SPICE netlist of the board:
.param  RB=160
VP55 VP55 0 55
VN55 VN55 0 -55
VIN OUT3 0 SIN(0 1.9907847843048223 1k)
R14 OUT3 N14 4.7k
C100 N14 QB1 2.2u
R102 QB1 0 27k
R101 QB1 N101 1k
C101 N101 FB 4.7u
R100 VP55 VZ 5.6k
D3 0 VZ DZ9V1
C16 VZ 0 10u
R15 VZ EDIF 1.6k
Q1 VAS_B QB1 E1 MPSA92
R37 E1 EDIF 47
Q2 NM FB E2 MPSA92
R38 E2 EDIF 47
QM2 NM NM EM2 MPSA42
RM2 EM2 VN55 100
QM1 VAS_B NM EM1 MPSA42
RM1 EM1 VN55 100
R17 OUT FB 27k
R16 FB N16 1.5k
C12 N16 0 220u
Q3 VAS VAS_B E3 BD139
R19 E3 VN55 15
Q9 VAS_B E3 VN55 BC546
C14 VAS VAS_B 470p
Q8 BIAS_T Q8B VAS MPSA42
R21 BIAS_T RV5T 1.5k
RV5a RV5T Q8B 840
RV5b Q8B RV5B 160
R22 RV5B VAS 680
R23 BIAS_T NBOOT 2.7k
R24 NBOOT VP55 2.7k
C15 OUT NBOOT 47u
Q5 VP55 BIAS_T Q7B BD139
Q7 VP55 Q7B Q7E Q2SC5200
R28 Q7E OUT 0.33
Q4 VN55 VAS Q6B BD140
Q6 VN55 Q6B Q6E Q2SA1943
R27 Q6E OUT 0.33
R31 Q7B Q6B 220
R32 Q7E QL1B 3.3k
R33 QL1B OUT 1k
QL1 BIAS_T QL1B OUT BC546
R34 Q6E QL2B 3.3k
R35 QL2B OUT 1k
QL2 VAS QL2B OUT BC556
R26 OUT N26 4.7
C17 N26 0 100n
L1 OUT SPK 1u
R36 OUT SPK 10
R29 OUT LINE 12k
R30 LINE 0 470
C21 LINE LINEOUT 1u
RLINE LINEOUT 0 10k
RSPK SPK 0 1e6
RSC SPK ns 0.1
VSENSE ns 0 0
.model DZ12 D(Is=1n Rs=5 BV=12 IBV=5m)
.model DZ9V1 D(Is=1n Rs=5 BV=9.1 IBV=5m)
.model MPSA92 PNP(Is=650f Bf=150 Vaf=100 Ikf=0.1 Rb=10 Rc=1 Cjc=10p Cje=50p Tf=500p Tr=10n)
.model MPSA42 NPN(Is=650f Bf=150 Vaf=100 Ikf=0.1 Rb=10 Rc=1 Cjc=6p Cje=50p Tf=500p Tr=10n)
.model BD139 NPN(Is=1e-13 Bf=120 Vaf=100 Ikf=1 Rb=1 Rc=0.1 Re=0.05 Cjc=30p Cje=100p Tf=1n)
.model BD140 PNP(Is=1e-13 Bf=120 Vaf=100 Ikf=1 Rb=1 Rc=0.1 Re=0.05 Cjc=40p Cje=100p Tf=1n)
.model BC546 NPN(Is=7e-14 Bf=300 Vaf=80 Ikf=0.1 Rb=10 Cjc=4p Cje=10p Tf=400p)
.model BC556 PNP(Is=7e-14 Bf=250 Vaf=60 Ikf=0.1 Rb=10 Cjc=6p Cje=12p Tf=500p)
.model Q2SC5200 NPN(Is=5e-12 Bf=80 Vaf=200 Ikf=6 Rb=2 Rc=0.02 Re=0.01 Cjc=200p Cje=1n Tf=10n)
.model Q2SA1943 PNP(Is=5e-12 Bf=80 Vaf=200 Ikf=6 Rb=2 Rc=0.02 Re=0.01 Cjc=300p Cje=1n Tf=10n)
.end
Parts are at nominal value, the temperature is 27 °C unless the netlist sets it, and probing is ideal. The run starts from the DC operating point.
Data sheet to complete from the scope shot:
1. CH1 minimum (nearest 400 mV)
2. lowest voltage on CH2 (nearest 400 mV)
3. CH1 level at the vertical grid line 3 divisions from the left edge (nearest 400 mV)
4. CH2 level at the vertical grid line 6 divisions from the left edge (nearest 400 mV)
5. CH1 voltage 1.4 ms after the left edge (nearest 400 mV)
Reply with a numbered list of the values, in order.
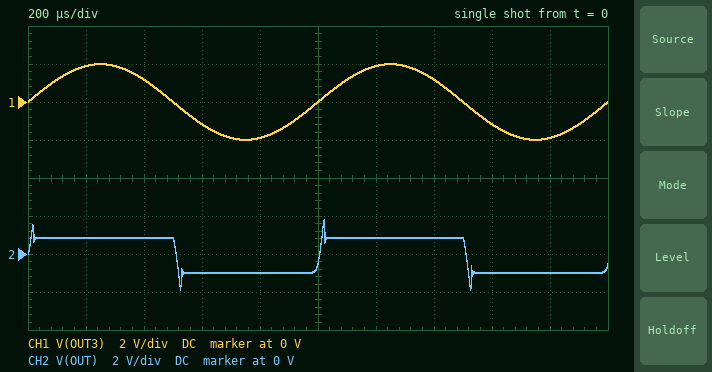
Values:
1. -2.0 V
2. -2.0 V
3. -1.2 V
4. 800 mV
5. 1.2 V
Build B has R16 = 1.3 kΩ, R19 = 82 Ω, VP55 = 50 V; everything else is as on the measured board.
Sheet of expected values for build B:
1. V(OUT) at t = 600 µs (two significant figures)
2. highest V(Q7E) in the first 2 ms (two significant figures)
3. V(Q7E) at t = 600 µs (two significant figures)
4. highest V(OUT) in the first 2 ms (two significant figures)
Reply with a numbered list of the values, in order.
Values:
1. 450 mV
2. 3.8 V
3. 1.9 V
4. 1.1 V
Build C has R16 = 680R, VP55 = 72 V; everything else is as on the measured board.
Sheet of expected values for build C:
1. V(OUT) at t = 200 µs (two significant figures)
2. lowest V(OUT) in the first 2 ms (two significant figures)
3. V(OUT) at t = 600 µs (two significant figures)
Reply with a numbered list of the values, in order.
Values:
1. 870 mV
2. -2.3 V
3. -990 mV
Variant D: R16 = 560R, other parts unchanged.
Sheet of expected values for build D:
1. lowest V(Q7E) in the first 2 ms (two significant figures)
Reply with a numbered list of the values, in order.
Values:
1. -2.3 V
